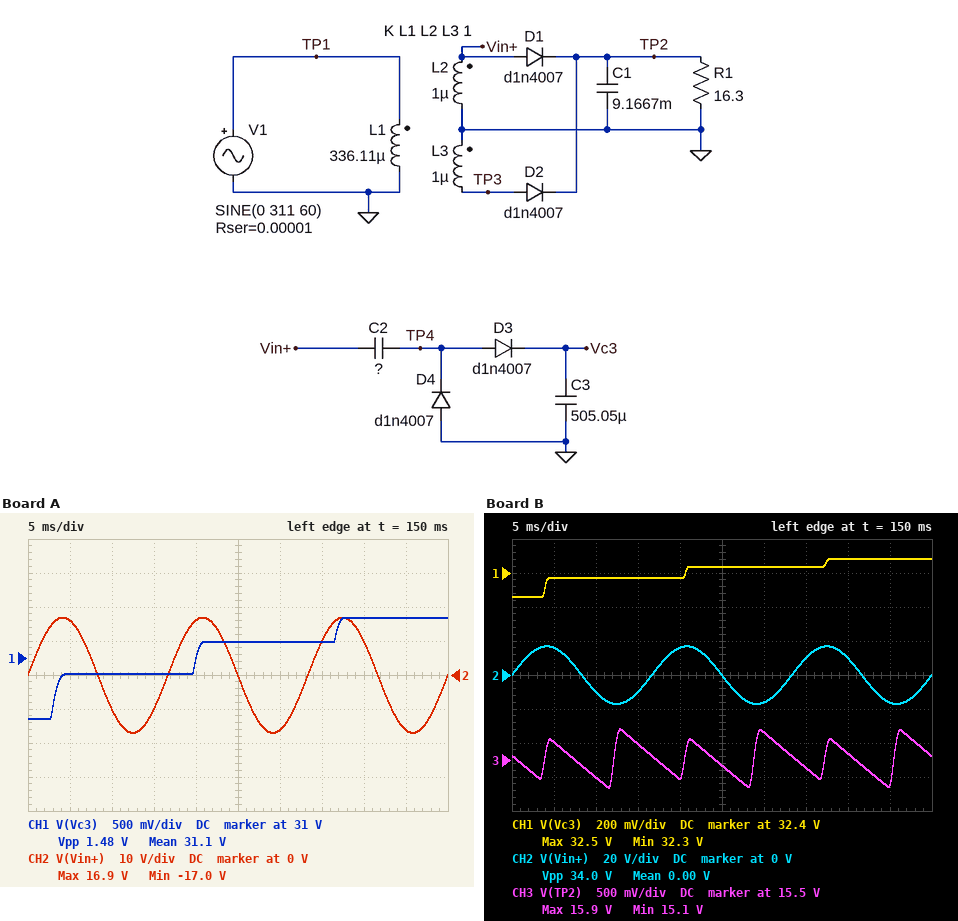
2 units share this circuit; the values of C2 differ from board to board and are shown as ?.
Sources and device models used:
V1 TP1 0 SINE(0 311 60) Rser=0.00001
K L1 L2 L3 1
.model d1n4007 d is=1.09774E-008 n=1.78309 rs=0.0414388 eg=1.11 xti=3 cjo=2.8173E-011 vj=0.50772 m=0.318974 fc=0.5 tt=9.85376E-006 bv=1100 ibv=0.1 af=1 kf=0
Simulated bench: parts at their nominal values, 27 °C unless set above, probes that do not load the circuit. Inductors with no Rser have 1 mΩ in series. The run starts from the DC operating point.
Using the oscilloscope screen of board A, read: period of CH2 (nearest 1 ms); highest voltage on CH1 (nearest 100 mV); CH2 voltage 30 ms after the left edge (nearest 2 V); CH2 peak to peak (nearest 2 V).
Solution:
17 ms
31.6 V
-16 V
34 V
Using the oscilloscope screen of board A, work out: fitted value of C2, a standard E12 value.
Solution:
180 µF
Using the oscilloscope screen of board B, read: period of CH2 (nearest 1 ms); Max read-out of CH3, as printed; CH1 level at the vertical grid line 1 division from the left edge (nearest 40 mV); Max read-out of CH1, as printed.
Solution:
17 ms
15.9 V
32.36 V
32.5 V
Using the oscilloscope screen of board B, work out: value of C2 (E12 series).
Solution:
390 µF
